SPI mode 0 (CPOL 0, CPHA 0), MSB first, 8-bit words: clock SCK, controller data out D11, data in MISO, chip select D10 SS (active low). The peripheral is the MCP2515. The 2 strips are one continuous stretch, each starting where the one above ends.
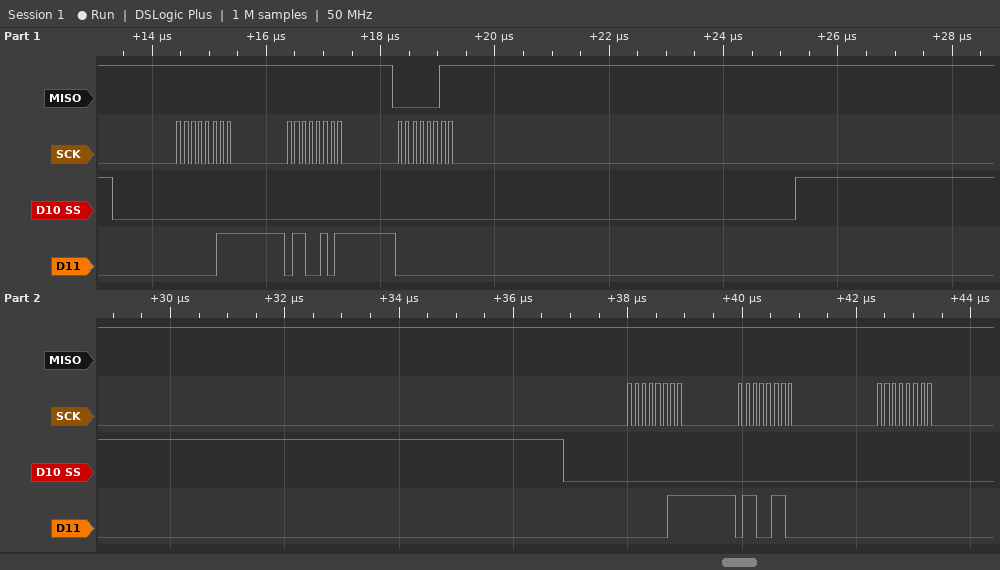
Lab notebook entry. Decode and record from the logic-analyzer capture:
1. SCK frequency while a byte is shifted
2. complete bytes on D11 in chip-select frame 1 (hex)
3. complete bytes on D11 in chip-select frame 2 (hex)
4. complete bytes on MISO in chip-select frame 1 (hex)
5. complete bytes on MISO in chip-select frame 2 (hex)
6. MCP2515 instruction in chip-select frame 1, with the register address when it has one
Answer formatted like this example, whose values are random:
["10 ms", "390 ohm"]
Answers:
["8 MHz", "03 65 00", "03 66 00", "FF FF 03", "FF FF FF", "READ 0x65"]
